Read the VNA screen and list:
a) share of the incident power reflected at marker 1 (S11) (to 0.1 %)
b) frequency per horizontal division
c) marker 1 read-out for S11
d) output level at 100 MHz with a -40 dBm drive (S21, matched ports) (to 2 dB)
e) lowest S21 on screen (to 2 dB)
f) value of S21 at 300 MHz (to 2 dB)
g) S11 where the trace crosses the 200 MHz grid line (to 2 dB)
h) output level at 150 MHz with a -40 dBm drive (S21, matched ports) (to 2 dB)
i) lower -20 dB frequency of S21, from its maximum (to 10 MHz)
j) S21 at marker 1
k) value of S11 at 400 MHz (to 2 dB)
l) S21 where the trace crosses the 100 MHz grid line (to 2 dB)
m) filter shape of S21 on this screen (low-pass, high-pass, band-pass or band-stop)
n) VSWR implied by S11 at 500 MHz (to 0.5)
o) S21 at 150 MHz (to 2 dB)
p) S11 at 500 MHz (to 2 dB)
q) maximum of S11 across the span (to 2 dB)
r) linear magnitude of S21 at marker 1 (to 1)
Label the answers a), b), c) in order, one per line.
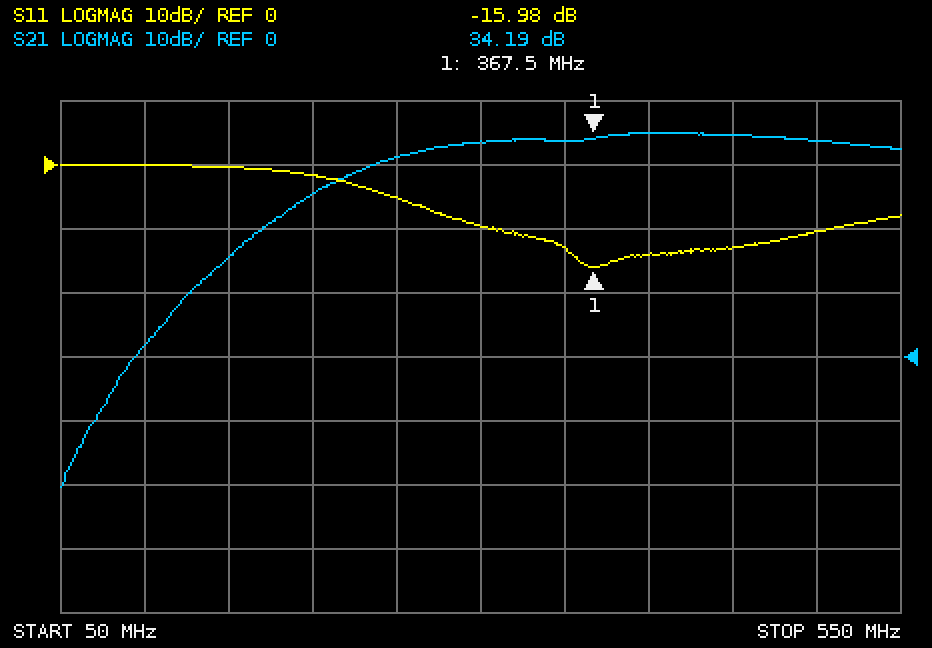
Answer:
a) 2.5 %
b) 50 MHz
c) -15.98 dB
d) -38 dBm
e) -20 dB
f) 34 dB
g) -2 dB
h) -24 dBm
i) 150 MHz
j) 34.19 dB
k) -14 dB
l) 2 dB
m) high-pass
n) 2.0
o) 16 dB
p) -10 dB
q) 0 dB
r) 51
